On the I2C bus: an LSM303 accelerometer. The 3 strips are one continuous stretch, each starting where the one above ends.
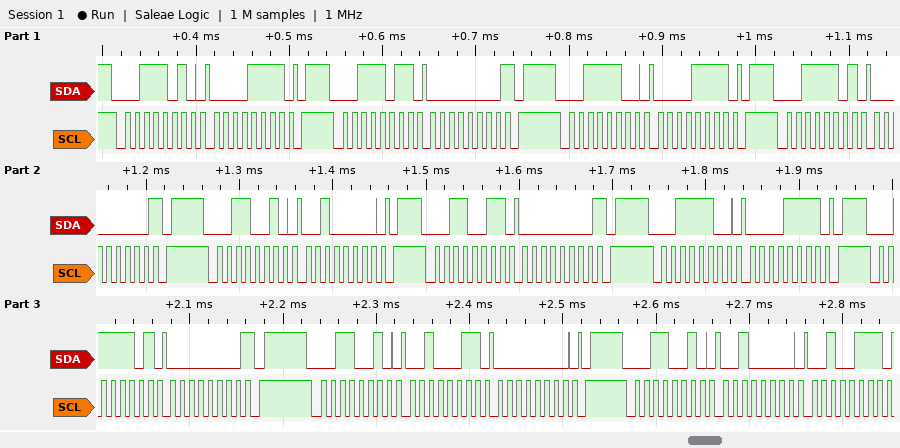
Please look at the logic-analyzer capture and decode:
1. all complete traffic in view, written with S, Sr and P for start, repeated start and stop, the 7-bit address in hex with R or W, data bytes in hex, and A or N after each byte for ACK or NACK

S 1DW A 0F A P S 1DR A 00 N P S 1EW A 0F A P S 1ER A 00 N P S 19W A 20 A P S 19R A 00 N P S 1EW A 0F A P S 1ER A 00 N P S 19W A 23 A 00 A P S 19W A 20 A 27 A
